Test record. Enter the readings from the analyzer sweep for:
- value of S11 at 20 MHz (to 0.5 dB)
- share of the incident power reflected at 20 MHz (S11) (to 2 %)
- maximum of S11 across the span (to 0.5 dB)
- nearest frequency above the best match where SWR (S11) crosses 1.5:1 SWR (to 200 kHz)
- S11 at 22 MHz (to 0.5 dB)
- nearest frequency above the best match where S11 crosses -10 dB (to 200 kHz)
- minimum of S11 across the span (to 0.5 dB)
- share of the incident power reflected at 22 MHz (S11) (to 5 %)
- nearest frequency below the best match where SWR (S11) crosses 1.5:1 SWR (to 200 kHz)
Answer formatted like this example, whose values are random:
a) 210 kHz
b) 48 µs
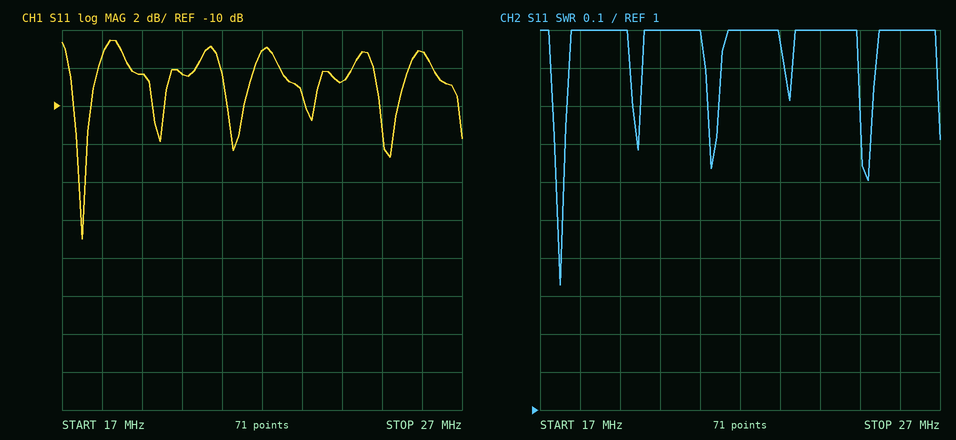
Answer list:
a) -8.5 dB
b) 14 %
c) -6.5 dB
d) 17.6 MHz
e) -7.0 dB
f) 17.8 MHz
g) -17.0 dB
h) 20 %
i) 17.4 MHz
